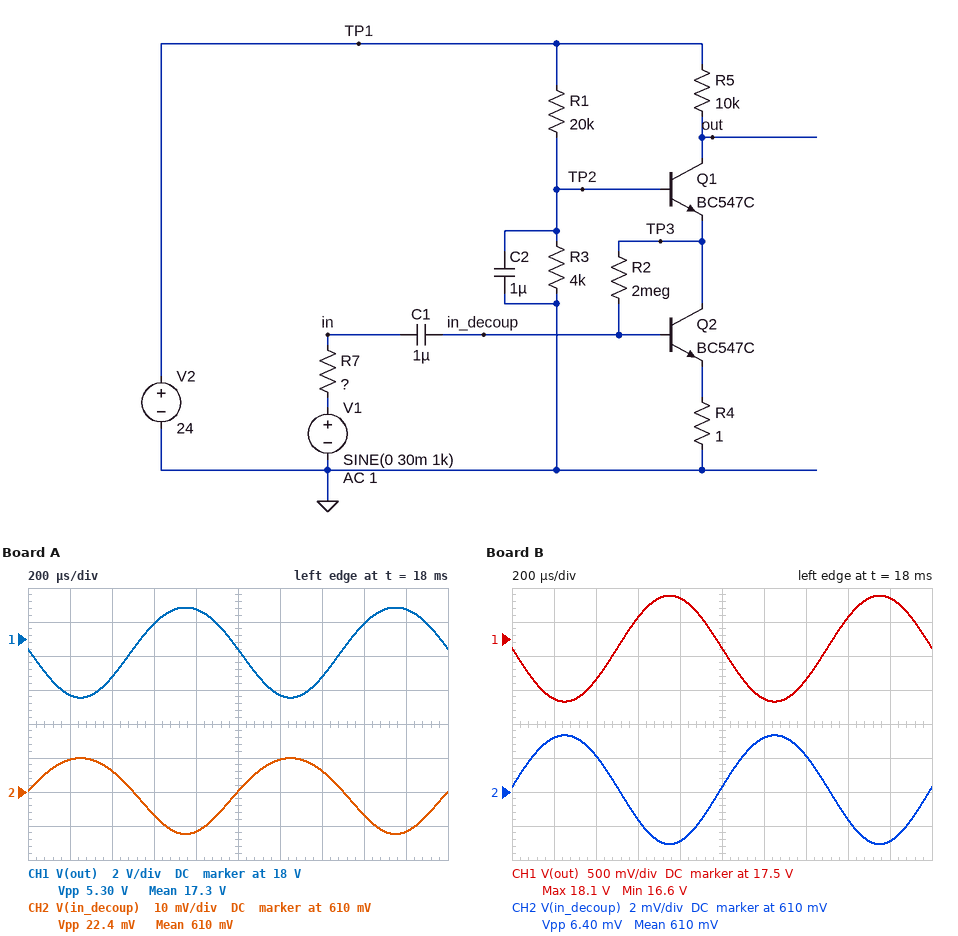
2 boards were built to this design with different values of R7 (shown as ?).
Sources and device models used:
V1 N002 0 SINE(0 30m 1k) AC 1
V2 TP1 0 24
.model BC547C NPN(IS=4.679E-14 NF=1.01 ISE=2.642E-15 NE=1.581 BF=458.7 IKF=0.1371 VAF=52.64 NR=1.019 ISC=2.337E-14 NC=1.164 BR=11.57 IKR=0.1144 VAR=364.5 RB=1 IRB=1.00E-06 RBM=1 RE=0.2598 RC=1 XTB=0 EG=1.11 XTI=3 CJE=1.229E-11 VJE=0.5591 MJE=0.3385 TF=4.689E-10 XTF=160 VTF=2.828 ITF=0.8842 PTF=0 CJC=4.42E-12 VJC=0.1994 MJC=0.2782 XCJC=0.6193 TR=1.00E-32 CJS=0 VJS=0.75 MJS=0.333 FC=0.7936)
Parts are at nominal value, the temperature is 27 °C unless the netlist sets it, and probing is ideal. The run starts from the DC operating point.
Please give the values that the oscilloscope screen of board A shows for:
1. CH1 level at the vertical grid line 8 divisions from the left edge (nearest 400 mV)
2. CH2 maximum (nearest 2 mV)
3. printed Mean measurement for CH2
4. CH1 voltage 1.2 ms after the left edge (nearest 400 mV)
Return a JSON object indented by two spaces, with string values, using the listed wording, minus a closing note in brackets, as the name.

{
  "CH1 level at the vertical grid line 8 divisions from the left edge": "18.8 V",
  "CH2 maximum": "620 mV",
  "printed Mean measurement for CH2": "610 mV",
  "CH1 voltage 1.2 ms after the left edge": "14.8 V"
}
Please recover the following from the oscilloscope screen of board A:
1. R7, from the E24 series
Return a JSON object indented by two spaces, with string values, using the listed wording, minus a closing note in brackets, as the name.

{
  "R7, from the E24 series": "33 kΩ"
}
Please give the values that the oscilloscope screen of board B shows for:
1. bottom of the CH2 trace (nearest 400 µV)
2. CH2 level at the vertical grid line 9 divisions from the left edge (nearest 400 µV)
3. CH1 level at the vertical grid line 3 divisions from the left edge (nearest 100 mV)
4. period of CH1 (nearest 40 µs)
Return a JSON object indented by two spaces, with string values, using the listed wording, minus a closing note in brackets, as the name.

{
  "bottom of the CH2 trace": "606.8 mV",
  "CH2 level at the vertical grid line 9 divisions from the left edge": "607.2 mV",
  "CH1 level at the vertical grid line 3 divisions from the left edge": "17.8 V",
  "period of CH1": "1.00 ms"
}
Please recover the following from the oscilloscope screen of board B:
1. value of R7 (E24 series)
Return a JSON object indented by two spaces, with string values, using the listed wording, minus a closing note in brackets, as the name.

{
  "value of R7": "160 kΩ"
}
